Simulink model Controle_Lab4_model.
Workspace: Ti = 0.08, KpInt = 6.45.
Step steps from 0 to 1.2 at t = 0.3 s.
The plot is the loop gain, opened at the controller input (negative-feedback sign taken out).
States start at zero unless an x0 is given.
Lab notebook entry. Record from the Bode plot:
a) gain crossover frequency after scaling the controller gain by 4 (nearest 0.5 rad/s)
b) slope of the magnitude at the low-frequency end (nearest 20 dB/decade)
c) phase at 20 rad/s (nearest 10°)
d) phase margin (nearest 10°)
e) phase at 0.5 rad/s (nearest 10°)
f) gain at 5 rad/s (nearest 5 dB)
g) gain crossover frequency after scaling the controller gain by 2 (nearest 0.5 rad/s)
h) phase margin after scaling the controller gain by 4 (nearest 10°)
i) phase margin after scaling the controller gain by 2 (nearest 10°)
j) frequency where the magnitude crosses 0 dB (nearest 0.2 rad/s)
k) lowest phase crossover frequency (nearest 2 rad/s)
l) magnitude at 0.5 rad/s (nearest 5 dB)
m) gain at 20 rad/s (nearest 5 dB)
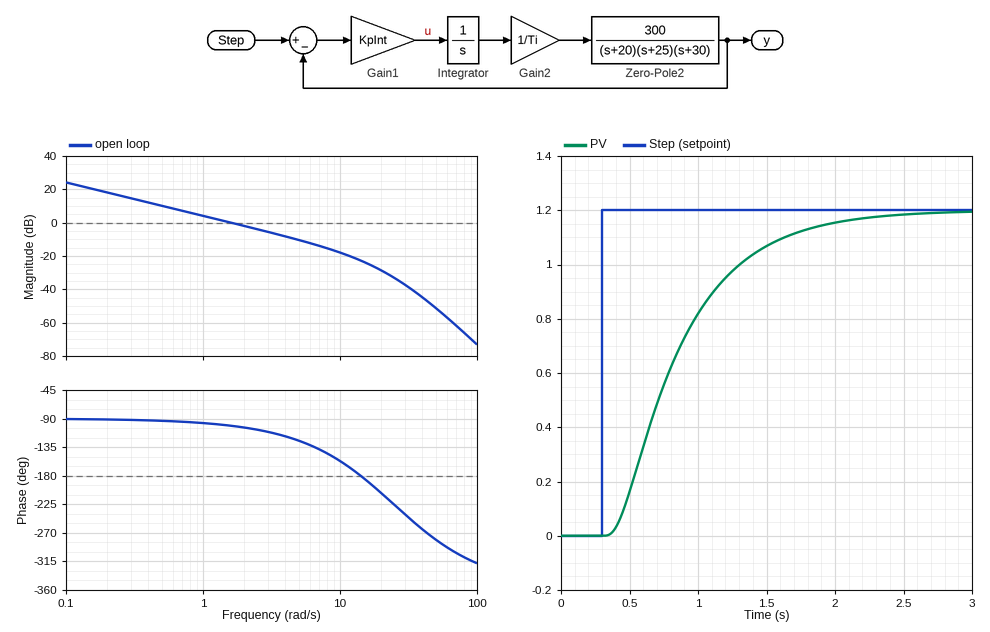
6.0 rad/s
-20 dB/decade
-210°
80°
-90°
-10 dB
3.0 rad/s
50°
70°
1.6 rad/s
14 rad/s
10 dB
-30 dB
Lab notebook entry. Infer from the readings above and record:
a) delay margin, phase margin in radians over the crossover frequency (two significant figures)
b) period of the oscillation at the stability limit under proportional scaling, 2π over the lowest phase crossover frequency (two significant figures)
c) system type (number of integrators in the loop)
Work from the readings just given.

0.87 s
0.45 s
1
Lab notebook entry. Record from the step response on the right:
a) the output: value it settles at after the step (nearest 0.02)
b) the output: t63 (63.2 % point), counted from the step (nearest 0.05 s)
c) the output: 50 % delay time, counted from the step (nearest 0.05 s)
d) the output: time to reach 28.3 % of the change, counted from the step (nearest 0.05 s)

1.20
0.65 s
0.50 s
0.30 s
